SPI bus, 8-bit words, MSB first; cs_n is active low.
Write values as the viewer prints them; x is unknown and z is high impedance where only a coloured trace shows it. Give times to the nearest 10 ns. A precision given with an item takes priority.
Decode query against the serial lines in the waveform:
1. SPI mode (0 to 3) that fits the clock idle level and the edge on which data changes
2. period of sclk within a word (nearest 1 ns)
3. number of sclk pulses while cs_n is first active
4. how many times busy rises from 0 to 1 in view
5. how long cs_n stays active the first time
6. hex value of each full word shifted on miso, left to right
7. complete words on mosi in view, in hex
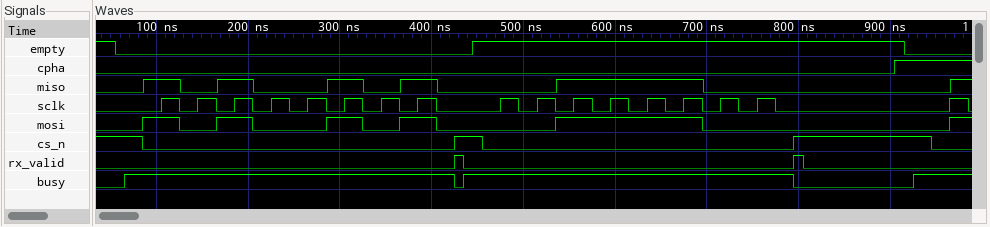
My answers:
0
40 ns
8
3
340 ns
A5, 3C
A5, 3C
